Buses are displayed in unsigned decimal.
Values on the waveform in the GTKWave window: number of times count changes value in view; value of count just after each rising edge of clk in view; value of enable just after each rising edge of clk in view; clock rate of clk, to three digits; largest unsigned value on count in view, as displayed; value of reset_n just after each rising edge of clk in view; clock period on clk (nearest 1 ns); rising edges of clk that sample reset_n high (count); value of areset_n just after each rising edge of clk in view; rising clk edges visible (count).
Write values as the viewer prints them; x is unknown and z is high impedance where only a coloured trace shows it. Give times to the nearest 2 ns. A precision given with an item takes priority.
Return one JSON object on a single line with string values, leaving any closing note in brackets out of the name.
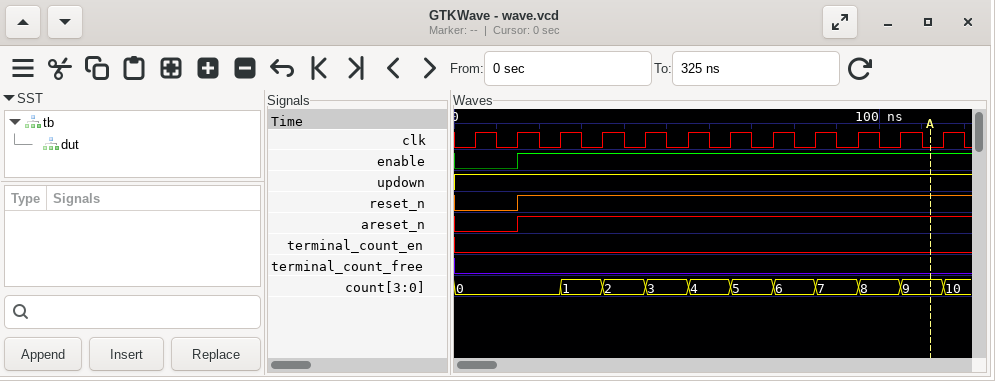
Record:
{"number of times count changes value in view": "10", "value of count just after each rising edge of clk in view": "0, 0, 1, 2, 3, 4, 5, 6, 7, 8, 9, 10", "value of enable just after each rising edge of clk in view": "0 1 1 1 1 1 1 1 1 1 1 1", "clock rate of clk, to three digits": "100 MHz", "largest unsigned value on count in view, as displayed": "10", "value of reset_n just after each rising edge of clk in view": "0 1 1 1 1 1 1 1 1 1 1 1", "clock period on clk": "10 ns", "rising edges of clk that sample reset_n high": "10", "value of areset_n just after each rising edge of clk in view": "0 1 1 1 1 1 1 1 1 1 1 1", "rising clk edges visible": "12"}
